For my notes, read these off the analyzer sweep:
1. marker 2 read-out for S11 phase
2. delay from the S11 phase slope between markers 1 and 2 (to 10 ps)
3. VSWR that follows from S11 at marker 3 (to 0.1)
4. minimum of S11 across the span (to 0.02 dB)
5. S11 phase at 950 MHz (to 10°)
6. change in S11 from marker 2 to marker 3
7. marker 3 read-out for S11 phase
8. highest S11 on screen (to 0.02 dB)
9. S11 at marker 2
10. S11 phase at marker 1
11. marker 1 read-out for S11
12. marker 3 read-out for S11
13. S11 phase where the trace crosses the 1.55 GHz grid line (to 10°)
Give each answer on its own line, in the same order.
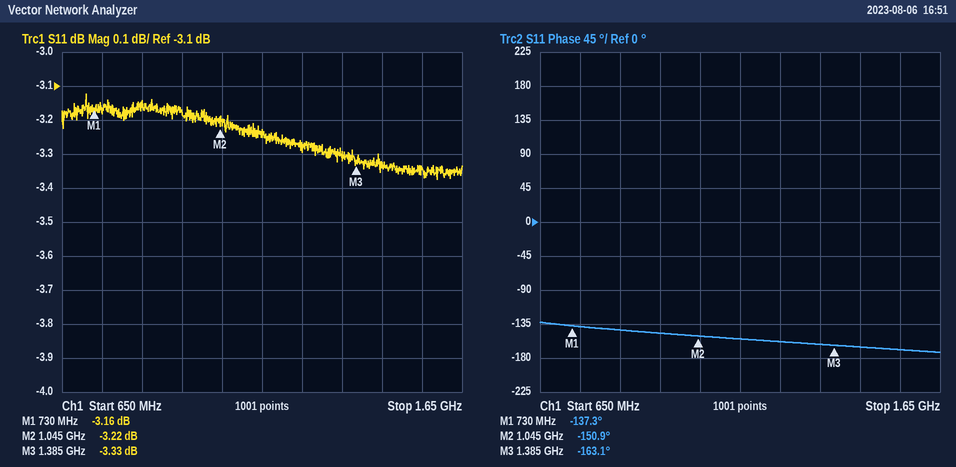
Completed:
-150.9°
120 ps
5.3
-3.38 dB
-150°
-0.11 dB
-163.1°
-3.12 dB
-3.22 dB
-137.3°
-3.16 dB
-3.33 dB
-170°
